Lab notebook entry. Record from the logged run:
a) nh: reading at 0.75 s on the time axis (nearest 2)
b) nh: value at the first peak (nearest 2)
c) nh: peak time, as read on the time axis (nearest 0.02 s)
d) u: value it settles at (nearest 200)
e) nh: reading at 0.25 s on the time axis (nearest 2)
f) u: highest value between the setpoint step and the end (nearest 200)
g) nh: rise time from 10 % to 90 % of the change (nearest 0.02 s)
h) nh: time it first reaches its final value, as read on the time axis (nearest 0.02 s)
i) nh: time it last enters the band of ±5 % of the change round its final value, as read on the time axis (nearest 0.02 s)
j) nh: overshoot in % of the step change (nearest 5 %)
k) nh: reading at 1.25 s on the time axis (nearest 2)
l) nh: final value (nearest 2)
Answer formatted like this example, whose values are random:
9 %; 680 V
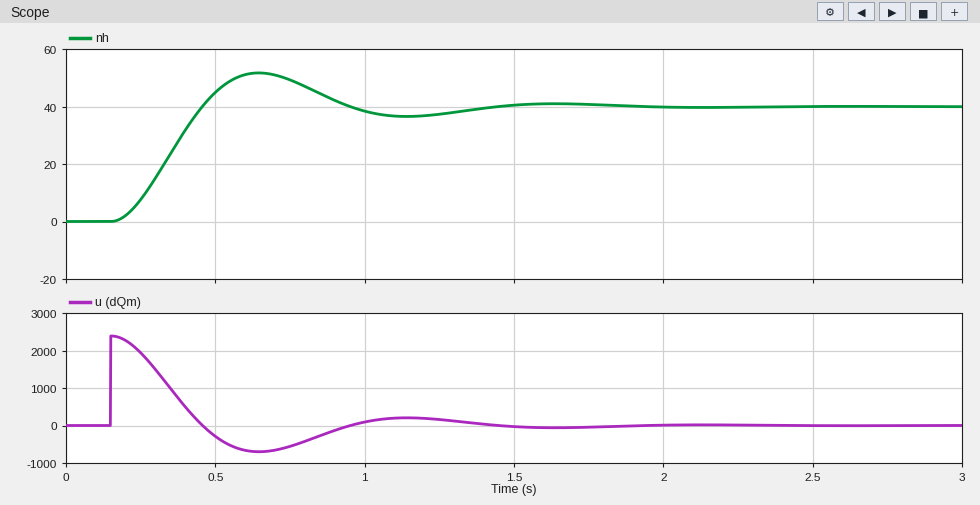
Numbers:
50; 52; 0.64 s; 0; 8; 2400; 0.20 s; 0.46 s; 1.30 s; 30 %; 38; 40
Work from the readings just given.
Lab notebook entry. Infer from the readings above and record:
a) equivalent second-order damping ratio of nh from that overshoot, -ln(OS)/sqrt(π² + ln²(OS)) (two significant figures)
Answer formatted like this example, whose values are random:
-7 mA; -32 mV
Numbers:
0.36
